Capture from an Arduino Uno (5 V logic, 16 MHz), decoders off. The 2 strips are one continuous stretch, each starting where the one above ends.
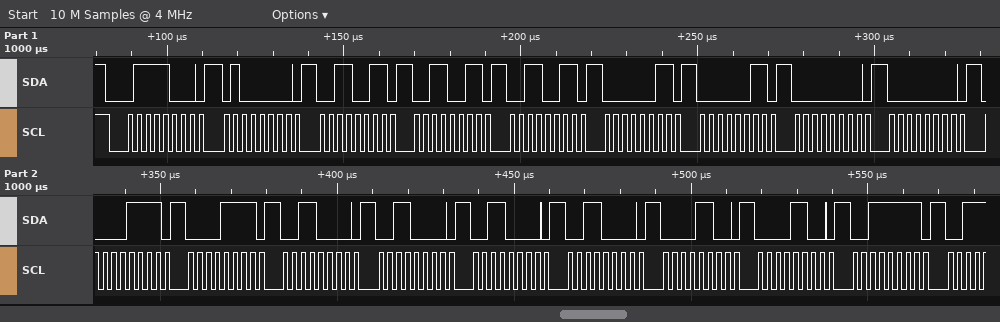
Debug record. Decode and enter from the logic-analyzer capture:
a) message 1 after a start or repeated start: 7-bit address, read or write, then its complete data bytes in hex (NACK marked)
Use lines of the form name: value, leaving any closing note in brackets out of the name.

message 1 after a start or repeated start: 7-bit address, read or write, then its complete data bytes in hex: 0x3C write: 40 33 33 33 03 03 00 00 0F 0F 30 30 30 30 0C 0C 3F
